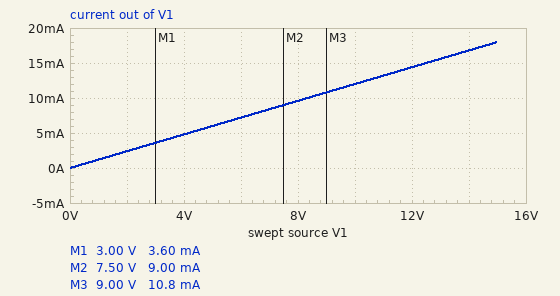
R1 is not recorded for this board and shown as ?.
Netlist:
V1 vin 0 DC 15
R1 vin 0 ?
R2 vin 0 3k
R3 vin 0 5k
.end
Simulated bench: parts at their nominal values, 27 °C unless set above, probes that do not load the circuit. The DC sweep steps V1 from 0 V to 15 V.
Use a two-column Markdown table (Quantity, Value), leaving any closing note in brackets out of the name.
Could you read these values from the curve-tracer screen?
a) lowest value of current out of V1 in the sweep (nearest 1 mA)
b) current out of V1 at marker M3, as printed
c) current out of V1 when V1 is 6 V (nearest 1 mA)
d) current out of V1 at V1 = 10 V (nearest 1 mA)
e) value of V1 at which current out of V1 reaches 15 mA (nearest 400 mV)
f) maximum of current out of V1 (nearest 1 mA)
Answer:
| Quantity | Value |
|---|---|
| lowest value of current out of V1 in the sweep | 0 A |
| current out of V1 at marker M3, as printed | 10.8 mA |
| current out of V1 when V1 is 6 V | 7 mA |
| current out of V1 at V1 = 10 V | 12 mA |
| value of V1 at which current out of V1 reaches 15 mA | 12.4 V |
| maximum of current out of V1 | 18 mA |
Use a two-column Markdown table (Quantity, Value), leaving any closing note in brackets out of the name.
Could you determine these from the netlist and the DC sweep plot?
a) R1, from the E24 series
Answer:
| Quantity | Value |
|---|---|
| R1, from the E24 series | 1.5 kΩ |
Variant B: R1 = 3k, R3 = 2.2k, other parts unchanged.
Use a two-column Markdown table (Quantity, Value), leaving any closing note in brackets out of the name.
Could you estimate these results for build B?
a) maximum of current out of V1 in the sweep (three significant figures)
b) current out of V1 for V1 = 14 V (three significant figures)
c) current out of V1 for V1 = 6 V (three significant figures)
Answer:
| Quantity | Value |
|---|---|
| maximum of current out of V1 in the sweep | 16.8 mA |
| current out of V1 for V1 = 14 V | 15.7 mA |
| current out of V1 for V1 = 6 V | 6.73 mA |
